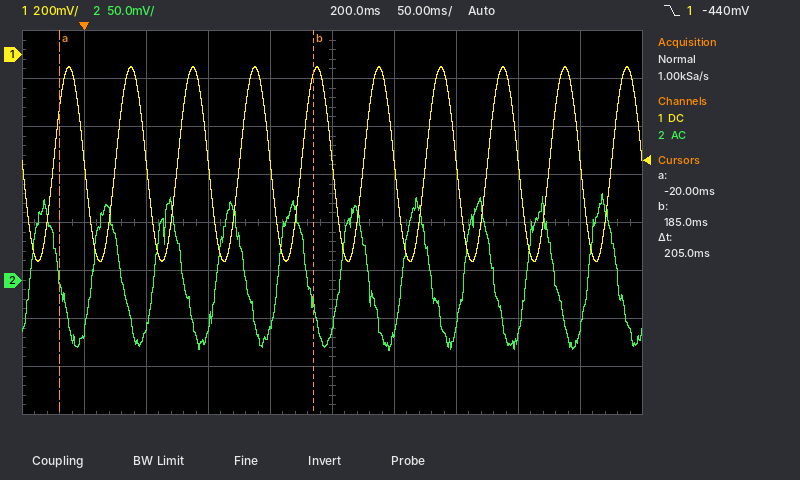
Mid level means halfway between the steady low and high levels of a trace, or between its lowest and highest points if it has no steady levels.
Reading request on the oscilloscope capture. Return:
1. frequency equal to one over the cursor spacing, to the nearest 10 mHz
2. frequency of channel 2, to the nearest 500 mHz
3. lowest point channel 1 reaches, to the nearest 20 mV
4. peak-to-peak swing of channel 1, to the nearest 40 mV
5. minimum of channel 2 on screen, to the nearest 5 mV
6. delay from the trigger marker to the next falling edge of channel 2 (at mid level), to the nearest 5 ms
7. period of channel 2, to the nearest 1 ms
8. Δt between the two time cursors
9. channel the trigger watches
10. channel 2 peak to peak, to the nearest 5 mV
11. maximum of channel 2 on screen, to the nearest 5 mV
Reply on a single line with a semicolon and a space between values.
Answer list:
4.88 Hz; 20.0 Hz; -860 mV; 800 mV; -75 mV; 30 ms; 50 ms; 205 ms; channel 1; 165 mV; 90 mV
